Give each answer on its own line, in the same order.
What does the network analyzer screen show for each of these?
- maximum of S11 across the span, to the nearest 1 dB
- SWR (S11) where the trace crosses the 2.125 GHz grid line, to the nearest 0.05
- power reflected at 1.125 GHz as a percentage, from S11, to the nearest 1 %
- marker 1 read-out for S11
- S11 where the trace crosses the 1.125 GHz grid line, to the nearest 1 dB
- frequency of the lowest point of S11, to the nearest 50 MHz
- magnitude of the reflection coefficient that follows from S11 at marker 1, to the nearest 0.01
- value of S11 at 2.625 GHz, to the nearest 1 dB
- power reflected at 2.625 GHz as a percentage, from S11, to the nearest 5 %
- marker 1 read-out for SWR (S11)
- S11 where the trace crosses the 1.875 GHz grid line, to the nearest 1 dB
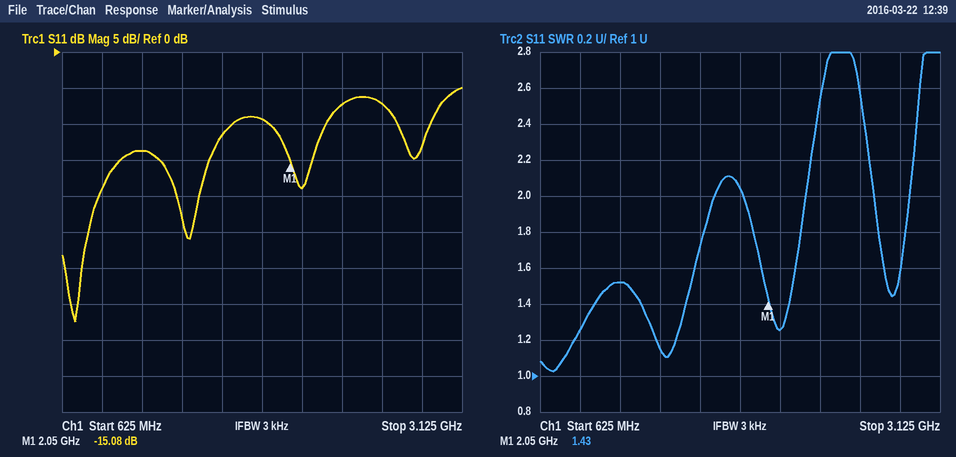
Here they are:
-5 dB
1.25
4 %
-15.08 dB
-14 dB
700 MHz
0.18
-7 dB
20 %
1.43
-9 dB
